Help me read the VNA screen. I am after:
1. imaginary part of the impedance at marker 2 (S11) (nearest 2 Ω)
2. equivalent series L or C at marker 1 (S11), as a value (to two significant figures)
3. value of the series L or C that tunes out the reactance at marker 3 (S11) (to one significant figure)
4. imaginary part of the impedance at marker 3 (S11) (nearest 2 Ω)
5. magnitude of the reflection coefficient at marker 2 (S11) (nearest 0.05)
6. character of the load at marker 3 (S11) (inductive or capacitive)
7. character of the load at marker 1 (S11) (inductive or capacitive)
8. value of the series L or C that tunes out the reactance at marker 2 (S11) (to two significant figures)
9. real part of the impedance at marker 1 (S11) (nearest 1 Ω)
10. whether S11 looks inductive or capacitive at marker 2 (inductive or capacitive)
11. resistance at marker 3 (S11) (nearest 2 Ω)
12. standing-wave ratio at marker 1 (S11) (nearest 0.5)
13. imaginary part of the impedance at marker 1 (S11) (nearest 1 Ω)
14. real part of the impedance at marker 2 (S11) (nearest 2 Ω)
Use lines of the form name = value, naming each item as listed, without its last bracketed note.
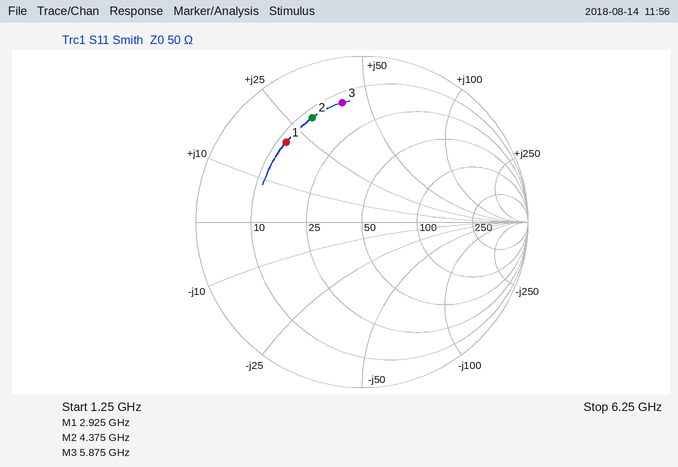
imaginary part of the impedance at marker 2 (S11) = +30 Ω
equivalent series L or C at marker 1 (S11), as a value = 1.1 nH
value of the series L or C that tunes out the reactance at marker 3 (S11) = 700 fF
imaginary part of the impedance at marker 3 (S11) = +40 Ω
magnitude of the reflection coefficient at marker 2 (S11) = 0.70
character of the load at marker 3 (S11) = inductive
character of the load at marker 1 (S11) = inductive
value of the series L or C that tunes out the reactance at marker 2 (S11) = 1.2 pF
real part of the impedance at marker 1 (S11) = 12 Ω
whether S11 looks inductive or capacitive at marker 2 = inductive
resistance at marker 3 (S11) = 14 Ω
standing-wave ratio at marker 1 (S11) = 5.0
imaginary part of the impedance at marker 1 (S11) = +20 Ω
real part of the impedance at marker 2 (S11) = 12 Ω
